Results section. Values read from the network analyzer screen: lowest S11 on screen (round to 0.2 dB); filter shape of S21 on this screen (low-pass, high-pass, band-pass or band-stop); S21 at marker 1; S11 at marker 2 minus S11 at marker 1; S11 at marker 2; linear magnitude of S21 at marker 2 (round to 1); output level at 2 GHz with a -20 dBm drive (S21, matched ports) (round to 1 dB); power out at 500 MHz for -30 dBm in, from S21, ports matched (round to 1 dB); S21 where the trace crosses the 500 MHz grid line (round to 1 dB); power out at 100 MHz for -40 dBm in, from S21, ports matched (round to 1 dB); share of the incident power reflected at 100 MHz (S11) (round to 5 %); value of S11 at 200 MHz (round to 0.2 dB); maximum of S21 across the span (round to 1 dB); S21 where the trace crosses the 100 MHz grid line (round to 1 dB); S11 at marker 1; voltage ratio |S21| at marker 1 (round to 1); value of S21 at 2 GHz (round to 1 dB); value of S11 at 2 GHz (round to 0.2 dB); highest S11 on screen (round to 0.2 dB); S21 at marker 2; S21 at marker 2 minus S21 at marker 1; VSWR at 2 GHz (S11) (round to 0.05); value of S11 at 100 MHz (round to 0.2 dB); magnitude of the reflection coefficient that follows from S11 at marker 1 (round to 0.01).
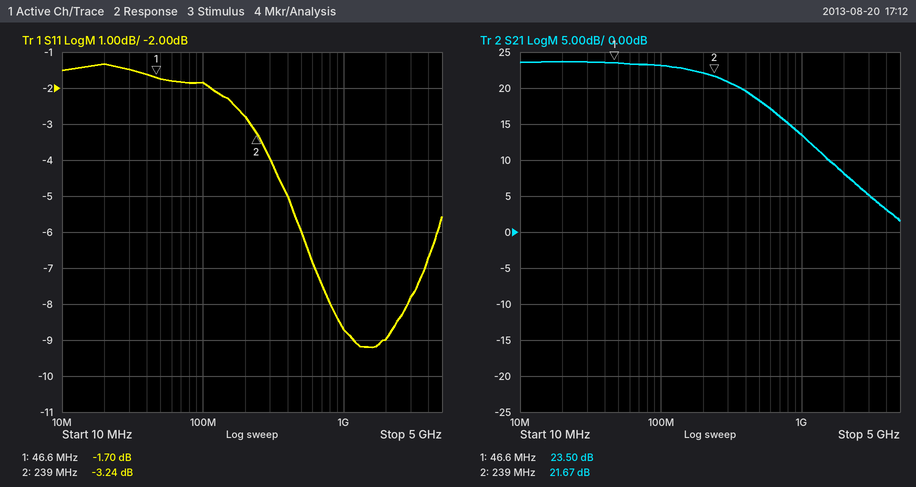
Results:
-9.2 dB
low-pass
23.50 dB
-1.54 dB
-3.24 dB
12
-12 dBm
-12 dBm
18 dB
-17 dBm
65 %
-2.8 dB
24 dB
23 dB
-1.70 dB
15
8 dB
-9.0 dB
-1.4 dB
21.67 dB
-1.83 dB
2.10
-1.8 dB
0.82
